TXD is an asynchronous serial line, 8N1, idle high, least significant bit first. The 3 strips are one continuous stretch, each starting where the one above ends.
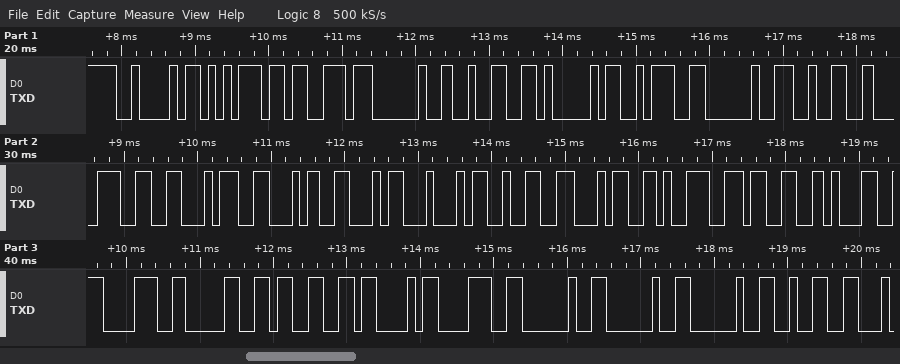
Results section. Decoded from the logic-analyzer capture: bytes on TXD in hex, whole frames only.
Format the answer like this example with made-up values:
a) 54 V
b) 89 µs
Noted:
a) 0x42 0x75 0x73 0x20 0x32 0x41 0x3A 0x20 0x32 0x38 0x46 0x46 0x46 0x44 0x32 0x34 0x39 0x33 0x31 0x38 0x30 0x33 0x43 0x38 0x20 0x20 0x20 0x32
